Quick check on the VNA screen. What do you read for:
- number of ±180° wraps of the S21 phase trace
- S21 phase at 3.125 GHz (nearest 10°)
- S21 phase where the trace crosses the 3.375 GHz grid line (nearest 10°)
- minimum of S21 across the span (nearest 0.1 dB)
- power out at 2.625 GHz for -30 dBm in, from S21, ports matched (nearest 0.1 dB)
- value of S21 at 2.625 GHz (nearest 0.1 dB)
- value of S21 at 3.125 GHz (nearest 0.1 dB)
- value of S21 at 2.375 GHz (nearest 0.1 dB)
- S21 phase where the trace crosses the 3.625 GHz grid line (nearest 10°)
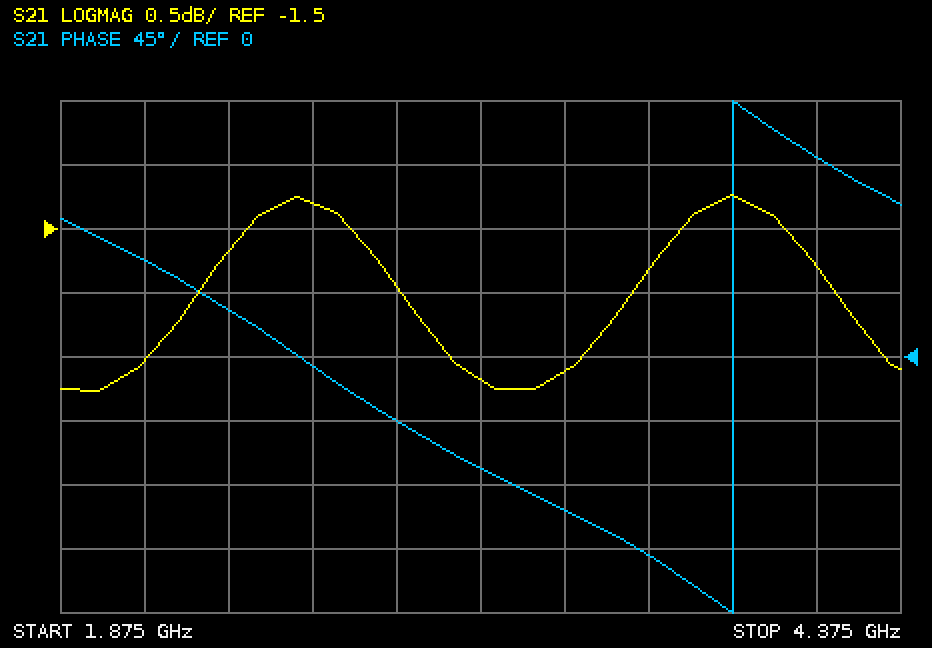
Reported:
1
-80°
-110°
-2.8 dB
-31.3 dBm
-1.3 dB
-2.7 dB
-1.7 dB
-140°
